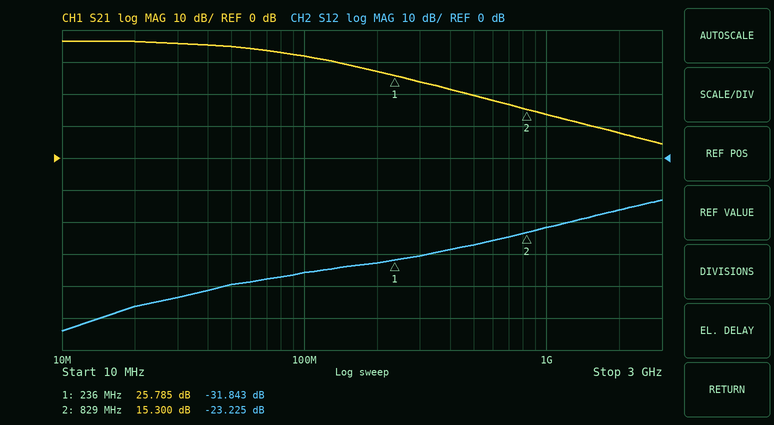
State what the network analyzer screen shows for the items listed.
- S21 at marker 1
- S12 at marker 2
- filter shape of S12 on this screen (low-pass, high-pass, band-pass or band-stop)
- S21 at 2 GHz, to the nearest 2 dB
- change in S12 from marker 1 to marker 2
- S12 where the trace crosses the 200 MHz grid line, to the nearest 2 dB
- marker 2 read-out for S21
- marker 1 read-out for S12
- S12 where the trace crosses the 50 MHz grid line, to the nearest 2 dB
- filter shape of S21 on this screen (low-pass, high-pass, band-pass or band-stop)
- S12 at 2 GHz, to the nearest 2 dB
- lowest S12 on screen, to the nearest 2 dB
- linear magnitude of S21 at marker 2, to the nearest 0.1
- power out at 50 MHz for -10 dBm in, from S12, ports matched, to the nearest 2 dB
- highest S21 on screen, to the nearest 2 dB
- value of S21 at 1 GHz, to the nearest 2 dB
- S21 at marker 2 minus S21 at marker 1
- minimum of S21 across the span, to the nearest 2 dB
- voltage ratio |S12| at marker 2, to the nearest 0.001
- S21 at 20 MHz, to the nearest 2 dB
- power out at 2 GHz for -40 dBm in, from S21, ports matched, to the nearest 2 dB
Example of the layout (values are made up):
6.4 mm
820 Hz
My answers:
25.785 dB
-23.225 dB
high-pass
8 dB
8.618 dB
-32 dB
15.300 dB
-31.843 dB
-40 dB
low-pass
-16 dB
-54 dB
5.8
-50 dBm
36 dB
14 dB
-10.485 dB
4 dB
0.069
36 dB
-32 dBm
